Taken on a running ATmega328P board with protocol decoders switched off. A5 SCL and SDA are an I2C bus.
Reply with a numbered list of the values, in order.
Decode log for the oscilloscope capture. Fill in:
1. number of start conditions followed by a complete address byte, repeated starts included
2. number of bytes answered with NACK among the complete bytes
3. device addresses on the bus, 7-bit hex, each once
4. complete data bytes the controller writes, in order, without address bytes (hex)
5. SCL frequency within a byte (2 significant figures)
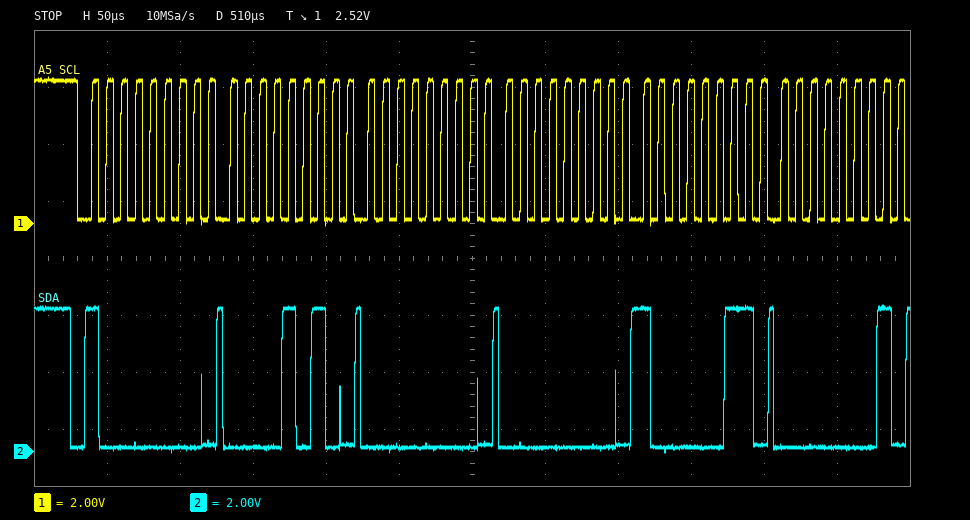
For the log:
1. 1
2. 0
3. 0x40
4. 0A 00 00 83 01
5. 100 kHz
